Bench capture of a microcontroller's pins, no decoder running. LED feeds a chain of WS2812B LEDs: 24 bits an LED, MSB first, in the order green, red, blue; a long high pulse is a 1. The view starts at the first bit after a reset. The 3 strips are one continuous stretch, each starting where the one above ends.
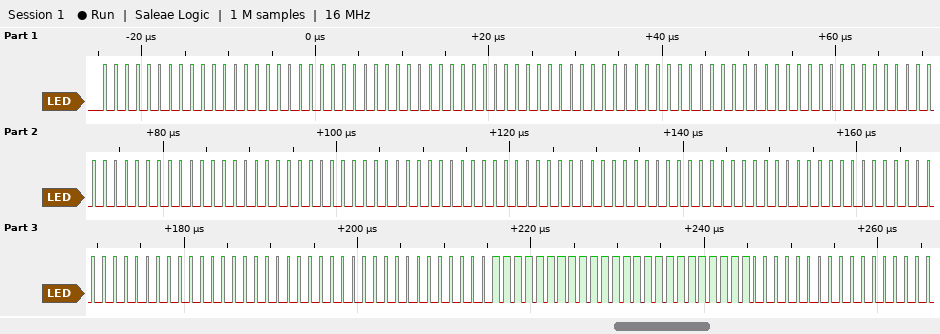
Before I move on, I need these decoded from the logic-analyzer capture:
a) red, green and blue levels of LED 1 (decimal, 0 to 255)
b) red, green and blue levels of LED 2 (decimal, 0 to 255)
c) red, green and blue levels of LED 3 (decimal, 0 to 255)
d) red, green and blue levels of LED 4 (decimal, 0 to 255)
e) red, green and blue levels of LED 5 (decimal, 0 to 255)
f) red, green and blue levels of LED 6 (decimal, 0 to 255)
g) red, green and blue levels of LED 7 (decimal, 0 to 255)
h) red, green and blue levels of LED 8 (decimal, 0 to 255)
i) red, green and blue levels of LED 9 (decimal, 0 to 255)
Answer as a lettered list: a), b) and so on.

a) 0, 0, 0
b) 0, 0, 0
c) 0, 0, 0
d) 0, 0, 0
e) 0, 0, 0
f) 0, 0, 0
g) 0, 0, 0
h) 0, 0, 0
i) 255, 255, 255
